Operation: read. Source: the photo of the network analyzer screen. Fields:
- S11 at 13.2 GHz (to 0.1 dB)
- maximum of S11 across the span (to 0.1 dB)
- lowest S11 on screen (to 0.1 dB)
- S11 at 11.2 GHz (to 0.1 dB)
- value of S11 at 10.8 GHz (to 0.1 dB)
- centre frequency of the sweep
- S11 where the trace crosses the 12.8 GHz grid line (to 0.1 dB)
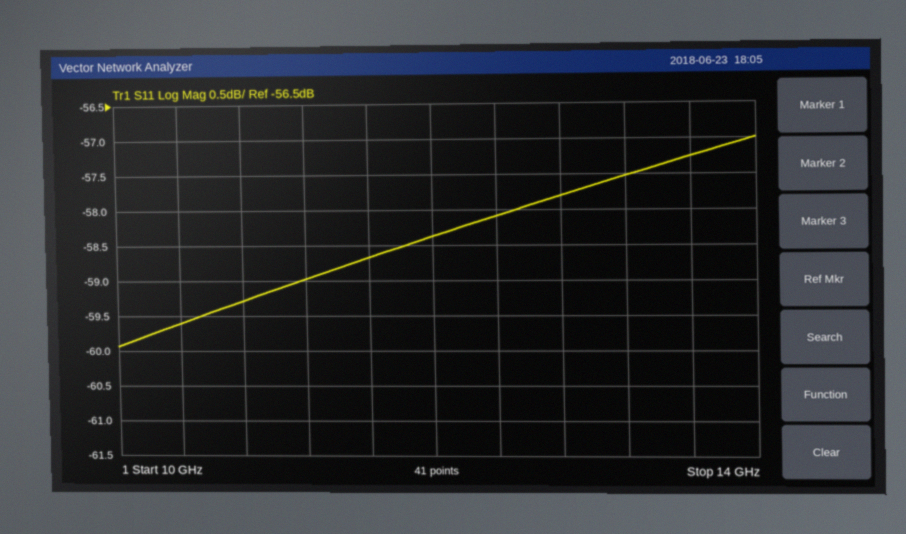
-57.5 dB
-57.0 dB
-59.9 dB
-59.0 dB
-59.3 dB
12 GHz
-57.8 dB
